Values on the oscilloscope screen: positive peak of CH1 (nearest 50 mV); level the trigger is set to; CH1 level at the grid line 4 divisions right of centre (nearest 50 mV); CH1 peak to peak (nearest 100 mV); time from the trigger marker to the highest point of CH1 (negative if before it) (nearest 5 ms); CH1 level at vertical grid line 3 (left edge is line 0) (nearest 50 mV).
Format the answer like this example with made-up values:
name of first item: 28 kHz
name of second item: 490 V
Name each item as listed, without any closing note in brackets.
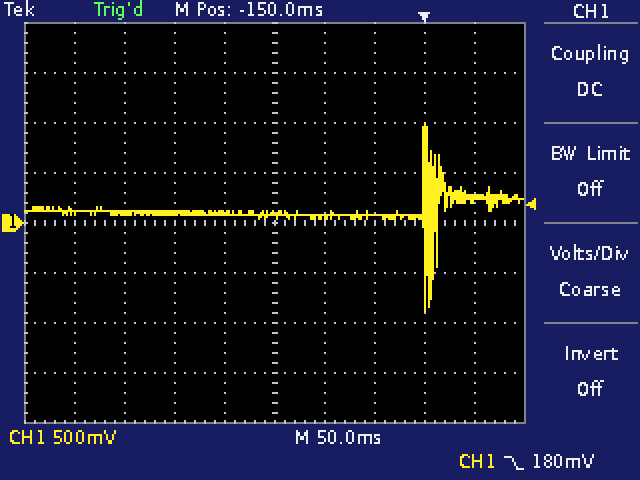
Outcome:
positive peak of CH1: 1.00 V
level the trigger is set to: 180 mV
CH1 level at the grid line 4 divisions right of centre: 250 mV
CH1 peak to peak: 1.90 V
time from the trigger marker to the highest point of CH1 (negative if before it): 0 ms
CH1 level at vertical grid line 3 (left edge is line 0): 100 mV
